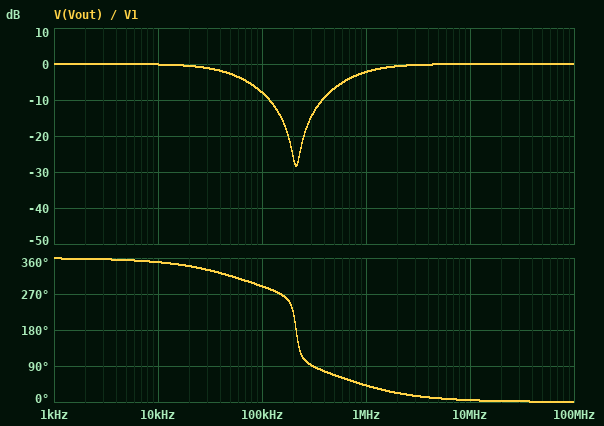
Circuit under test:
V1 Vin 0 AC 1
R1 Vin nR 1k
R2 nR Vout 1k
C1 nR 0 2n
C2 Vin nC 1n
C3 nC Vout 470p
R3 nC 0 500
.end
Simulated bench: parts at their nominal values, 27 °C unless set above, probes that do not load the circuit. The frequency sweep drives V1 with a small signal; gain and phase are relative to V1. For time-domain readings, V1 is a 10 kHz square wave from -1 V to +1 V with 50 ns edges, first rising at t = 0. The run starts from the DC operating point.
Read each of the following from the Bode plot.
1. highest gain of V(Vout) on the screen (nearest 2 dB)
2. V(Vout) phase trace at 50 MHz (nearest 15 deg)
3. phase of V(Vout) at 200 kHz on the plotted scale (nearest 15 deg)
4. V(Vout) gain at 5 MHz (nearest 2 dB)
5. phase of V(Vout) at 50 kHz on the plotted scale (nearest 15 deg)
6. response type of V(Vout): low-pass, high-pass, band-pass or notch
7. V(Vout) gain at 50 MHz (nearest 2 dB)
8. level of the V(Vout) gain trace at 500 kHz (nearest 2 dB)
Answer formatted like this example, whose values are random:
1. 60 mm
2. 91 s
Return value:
1. 0 dB
2. 0 deg
3. 225 deg
4. 0 dB
5. 315 deg
6. notch
7. 0 dB
8. -6 dB
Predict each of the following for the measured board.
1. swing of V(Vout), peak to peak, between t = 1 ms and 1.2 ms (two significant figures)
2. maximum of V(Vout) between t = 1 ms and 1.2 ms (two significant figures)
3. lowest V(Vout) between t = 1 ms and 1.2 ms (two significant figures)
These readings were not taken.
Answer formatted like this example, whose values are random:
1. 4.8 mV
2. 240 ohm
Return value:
1. 2.0 V
2. 1.0 V
3. -1.0 V
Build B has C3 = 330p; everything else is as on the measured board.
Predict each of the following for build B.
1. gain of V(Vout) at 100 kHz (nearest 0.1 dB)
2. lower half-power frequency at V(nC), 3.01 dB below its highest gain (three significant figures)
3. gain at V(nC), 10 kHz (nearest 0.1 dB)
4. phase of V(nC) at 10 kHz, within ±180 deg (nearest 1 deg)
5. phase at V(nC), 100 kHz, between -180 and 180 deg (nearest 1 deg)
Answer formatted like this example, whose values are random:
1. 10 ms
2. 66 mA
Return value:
1. -6.7 dB
2. 504 kHz
3. -27.6 dB
4. 85 deg
5. 60 deg
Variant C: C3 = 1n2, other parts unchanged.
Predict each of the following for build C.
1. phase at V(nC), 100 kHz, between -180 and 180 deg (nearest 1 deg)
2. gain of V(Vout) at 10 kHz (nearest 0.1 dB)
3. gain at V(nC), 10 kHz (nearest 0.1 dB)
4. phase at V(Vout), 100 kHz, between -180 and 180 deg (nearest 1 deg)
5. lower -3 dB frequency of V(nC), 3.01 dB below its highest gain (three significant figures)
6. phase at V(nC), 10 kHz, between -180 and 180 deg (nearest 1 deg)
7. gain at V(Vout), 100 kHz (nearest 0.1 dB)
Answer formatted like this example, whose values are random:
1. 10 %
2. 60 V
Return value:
1. 43 deg
2. -0.3 dB
3. -23.5 dB
4. -75 deg
5. 553 kHz
6. 78 deg
7. -14.3 dB
